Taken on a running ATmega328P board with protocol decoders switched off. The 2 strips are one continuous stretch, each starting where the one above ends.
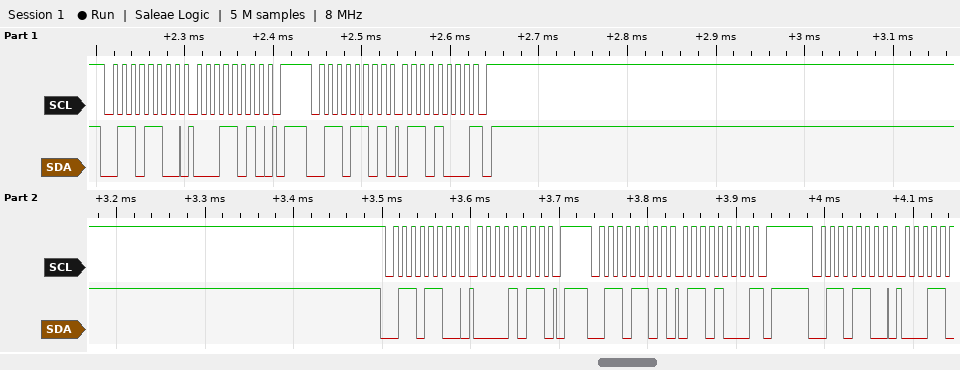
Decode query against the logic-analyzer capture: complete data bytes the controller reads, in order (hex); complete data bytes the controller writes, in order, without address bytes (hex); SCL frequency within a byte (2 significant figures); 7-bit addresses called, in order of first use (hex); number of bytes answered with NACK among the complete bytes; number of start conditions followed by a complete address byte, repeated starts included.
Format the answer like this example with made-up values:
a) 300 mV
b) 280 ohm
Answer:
a) 68 68
b) 1A 0B
c) 100 kHz
d) 0x36
e) 2
f) 5
